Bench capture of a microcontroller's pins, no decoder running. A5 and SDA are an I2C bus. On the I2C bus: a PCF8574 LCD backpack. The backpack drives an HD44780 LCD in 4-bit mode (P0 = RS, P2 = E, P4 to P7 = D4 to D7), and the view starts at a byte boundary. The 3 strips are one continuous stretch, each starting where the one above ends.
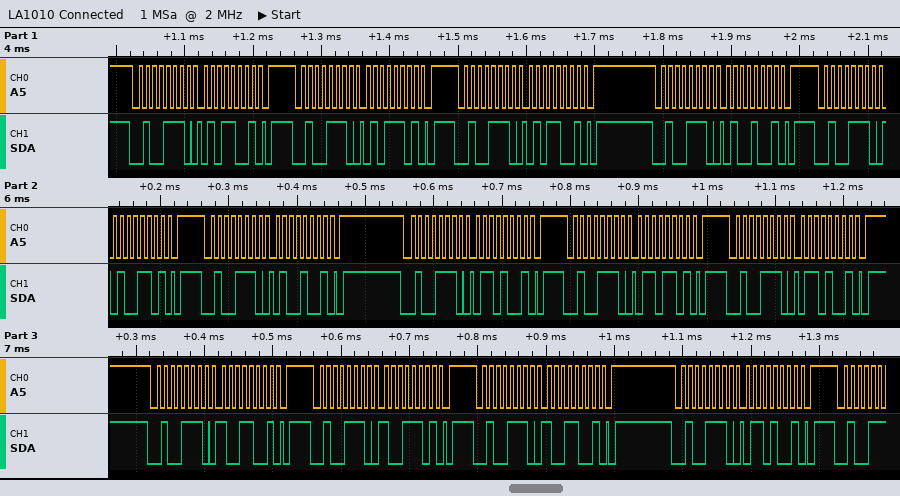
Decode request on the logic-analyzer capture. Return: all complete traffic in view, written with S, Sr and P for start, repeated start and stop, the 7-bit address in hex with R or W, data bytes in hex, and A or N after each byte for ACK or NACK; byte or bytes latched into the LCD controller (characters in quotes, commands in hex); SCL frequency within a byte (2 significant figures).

S 27W A 59 A P S 27W A 5D A P S 27W A 59 A P S 27W A 49 A P S 27W A 4D A P S 27W A 49 A P S 27W A 69 A P S 27W A 6D A P S 27W A 69 A P S 27W A 99 A P S 27W A 9D A P S 27W A 99 A P S 27W A 69 A P
'T' 'i'
100 kHz
